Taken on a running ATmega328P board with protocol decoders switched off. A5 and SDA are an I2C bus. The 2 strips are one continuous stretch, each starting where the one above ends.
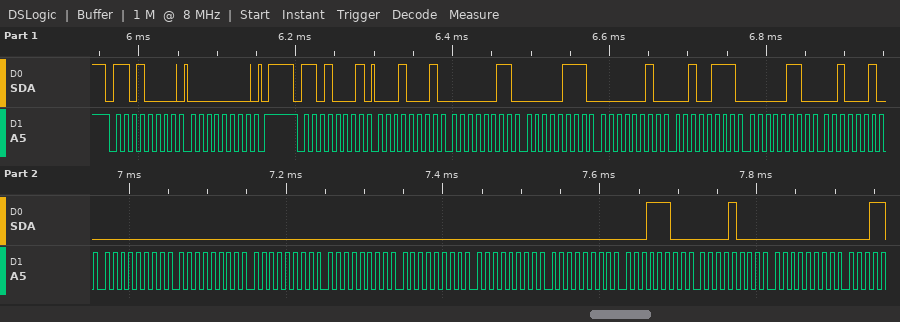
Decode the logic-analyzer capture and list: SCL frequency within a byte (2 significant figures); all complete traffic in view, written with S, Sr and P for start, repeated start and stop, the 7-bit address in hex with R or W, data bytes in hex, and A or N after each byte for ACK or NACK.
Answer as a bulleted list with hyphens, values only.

- 100 kHz
- S 68W A 00 A P S 68R A 11 A 03 A 07 A 02 A 27 A 06 A 22 A 00 A 00 A 00 A 00 A 00 A 00 A 00 A 1C A 08 A 00 A
